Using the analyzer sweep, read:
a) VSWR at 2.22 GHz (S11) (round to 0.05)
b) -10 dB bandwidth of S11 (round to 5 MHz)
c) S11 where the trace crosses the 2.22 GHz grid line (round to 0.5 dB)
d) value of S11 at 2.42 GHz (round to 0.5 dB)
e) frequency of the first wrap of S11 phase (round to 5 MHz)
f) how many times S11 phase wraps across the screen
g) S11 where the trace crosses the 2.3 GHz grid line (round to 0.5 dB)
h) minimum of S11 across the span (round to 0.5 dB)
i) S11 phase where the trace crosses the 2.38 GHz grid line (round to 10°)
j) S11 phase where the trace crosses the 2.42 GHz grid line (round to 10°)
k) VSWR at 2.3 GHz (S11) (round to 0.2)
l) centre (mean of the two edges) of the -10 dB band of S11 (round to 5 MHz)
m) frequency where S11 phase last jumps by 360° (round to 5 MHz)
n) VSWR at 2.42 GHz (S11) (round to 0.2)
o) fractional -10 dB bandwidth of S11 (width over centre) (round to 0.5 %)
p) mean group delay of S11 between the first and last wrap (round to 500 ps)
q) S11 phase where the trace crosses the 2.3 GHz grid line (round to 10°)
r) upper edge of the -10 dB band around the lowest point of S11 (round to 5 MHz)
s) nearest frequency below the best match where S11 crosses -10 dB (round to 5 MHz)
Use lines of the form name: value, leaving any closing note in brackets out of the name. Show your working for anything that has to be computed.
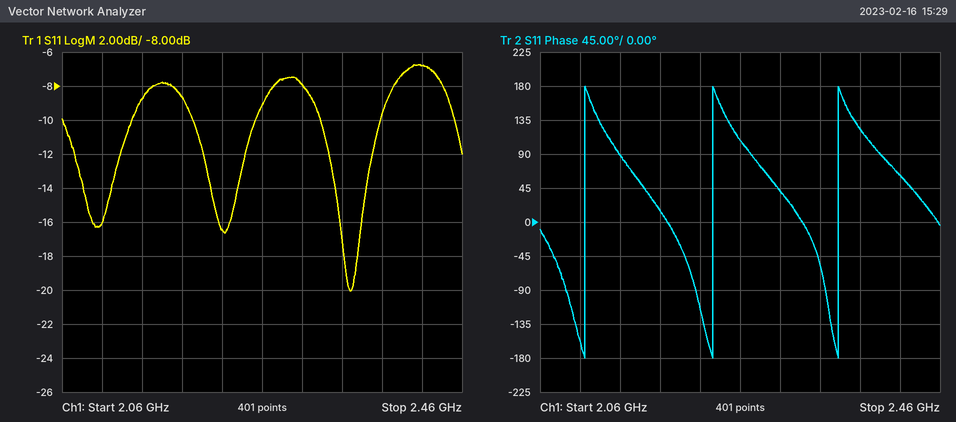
VSWR at 2.22 GHz (S11): |Γ| = 10^(-16.5/20) = 0.1496; VSWR = (1 + 0.1496)/(1 − 0.1496) ≈ 1.35
-10 dB bandwidth of S11: 2.380 GHz − 2.320 GHz = 60 MHz
S11 where the trace crosses the 2.22 GHz grid line: -16.5 dB
value of S11 at 2.42 GHz: -7.0 dB
frequency of the first wrap of S11 phase: 2.105 GHz
how many times S11 phase wraps across the screen: 3
S11 where the trace crosses the 2.3 GHz grid line: -8.0 dB
minimum of S11 across the span: -20.0 dB
S11 phase where the trace crosses the 2.38 GHz grid line: 120°
S11 phase where the trace crosses the 2.42 GHz grid line: 60°
VSWR at 2.3 GHz (S11): |Γ| = 10^(-8/20) = 0.3981; VSWR = (1 + 0.3981)/(1 − 0.3981) ≈ 2.32, so 2.4 to the nearest 0.2
centre (mean of the two edges) of the -10 dB band of S11: 2.350 GHz
frequency where S11 phase last jumps by 360°: 2.360 GHz
VSWR at 2.42 GHz (S11): |Γ| = 10^(-7/20) = 0.4467; VSWR = (1 + 0.4467)/(1 − 0.4467) ≈ 2.6
fractional -10 dB bandwidth of S11 (width over centre): 60 MHz / 2.35 GHz ≈ 2.5 %
mean group delay of S11 between the first and last wrap: 2 cycles / (2.360 GHz − 2.105 GHz) ≈ 7.84 ns, so 8.0 ns to the nearest 500 ps
S11 phase where the trace crosses the 2.3 GHz grid line: 40°
upper edge of the -10 dB band around the lowest point of S11: 2.380 GHz
nearest frequency below the best match where S11 crosses -10 dB: 2.320 GHz
